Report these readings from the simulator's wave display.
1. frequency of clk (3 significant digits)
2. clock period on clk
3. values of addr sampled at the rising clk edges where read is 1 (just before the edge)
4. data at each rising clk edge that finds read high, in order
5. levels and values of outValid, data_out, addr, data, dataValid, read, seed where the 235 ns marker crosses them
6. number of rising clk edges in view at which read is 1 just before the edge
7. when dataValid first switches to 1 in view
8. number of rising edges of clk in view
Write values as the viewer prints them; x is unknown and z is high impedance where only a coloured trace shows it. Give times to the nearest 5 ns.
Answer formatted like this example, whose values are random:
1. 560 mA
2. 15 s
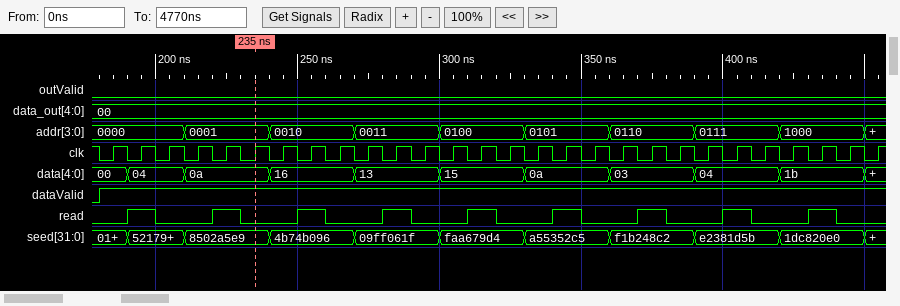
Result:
1. 100 MHz
2. 10 ns
3. 0000, 0001, 0010, 0011, 0100, 0101, 0110, 0111, 1000
4. 04, 0a, 16, 13, 15, 0a, 03, 04, 1b
5. outValid=0, data_out=00, addr=0001, data=0a, dataValid=1, read=0, seed=8502a5e9
6. 9
7. 180 ns
8. 28
